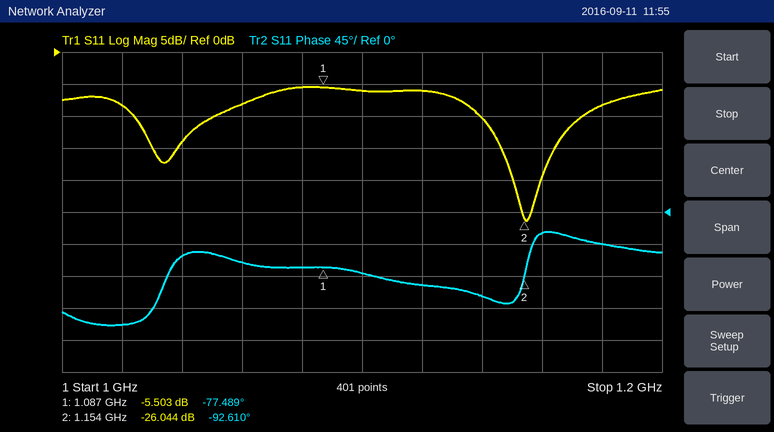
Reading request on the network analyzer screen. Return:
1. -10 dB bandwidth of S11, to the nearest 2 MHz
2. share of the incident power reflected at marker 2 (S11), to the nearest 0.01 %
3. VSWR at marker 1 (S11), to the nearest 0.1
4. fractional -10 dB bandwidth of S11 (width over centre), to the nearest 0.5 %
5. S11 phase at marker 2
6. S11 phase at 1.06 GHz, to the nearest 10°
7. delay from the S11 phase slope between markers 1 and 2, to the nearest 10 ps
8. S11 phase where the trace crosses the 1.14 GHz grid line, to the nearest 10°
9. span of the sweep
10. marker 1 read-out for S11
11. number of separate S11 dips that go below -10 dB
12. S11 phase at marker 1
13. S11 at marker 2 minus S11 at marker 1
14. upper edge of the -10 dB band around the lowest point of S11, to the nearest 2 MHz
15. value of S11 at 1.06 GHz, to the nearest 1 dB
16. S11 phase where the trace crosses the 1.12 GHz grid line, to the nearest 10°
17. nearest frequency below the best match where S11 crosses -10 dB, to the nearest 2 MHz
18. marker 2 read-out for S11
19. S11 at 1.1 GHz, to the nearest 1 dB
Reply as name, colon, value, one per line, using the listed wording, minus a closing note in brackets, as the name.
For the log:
-10 dB bandwidth of S11, to the nearest 2 MHz: 34 MHz
share of the incident power reflected at marker 2 (S11), to the nearest 0.01 %: 0.25 %
VSWR at marker 1 (S11), to the nearest 0.1: 3.3
fractional -10 dB bandwidth of S11 (width over centre), to the nearest 0.5 %: 3.0 %
S11 phase at marker 2: -92.610°
S11 phase at 1.06 GHz, to the nearest 10°: -70°
delay from the S11 phase slope between markers 1 and 2, to the nearest 10 ps: 630 ps
S11 phase where the trace crosses the 1.14 GHz grid line, to the nearest 10°: -120°
span of the sweep: 200 MHz
marker 1 read-out for S11: -5.503 dB
number of separate S11 dips that go below -10 dB: 2
S11 phase at marker 1: -77.489°
S11 at marker 2 minus S11 at marker 1: -20.541 dB
upper edge of the -10 dB band around the lowest point of S11, to the nearest 2 MHz: 1.174 GHz
value of S11 at 1.06 GHz, to the nearest 1 dB: -8 dB
S11 phase where the trace crosses the 1.12 GHz grid line, to the nearest 10°: -100°
nearest frequency below the best match where S11 crosses -10 dB, to the nearest 2 MHz: 1.140 GHz
marker 2 read-out for S11: -26.044 dB
S11 at 1.1 GHz, to the nearest 1 dB: -6 dB
